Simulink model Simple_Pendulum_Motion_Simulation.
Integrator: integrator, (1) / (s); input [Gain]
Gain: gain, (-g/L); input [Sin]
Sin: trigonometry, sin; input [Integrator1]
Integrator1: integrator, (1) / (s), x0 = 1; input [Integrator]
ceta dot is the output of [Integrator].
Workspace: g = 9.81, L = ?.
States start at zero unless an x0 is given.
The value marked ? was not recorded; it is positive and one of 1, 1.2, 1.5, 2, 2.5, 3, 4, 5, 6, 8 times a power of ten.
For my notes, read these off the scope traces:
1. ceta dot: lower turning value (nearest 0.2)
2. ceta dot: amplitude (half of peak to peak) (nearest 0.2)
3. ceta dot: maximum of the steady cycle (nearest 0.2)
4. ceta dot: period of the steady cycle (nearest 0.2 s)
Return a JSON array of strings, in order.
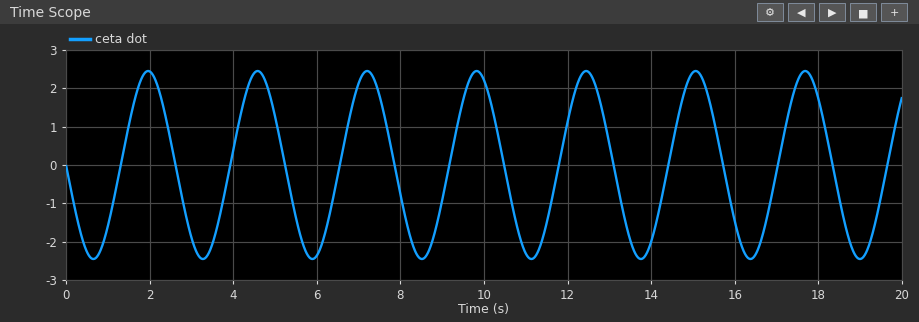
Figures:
["-2.4", "2.4", "2.4", "2.6 s"]
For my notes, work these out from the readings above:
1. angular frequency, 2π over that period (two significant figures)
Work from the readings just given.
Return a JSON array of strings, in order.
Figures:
["2.4 rad/s"]
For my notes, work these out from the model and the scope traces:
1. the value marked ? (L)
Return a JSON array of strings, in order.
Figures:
["1.5"]
